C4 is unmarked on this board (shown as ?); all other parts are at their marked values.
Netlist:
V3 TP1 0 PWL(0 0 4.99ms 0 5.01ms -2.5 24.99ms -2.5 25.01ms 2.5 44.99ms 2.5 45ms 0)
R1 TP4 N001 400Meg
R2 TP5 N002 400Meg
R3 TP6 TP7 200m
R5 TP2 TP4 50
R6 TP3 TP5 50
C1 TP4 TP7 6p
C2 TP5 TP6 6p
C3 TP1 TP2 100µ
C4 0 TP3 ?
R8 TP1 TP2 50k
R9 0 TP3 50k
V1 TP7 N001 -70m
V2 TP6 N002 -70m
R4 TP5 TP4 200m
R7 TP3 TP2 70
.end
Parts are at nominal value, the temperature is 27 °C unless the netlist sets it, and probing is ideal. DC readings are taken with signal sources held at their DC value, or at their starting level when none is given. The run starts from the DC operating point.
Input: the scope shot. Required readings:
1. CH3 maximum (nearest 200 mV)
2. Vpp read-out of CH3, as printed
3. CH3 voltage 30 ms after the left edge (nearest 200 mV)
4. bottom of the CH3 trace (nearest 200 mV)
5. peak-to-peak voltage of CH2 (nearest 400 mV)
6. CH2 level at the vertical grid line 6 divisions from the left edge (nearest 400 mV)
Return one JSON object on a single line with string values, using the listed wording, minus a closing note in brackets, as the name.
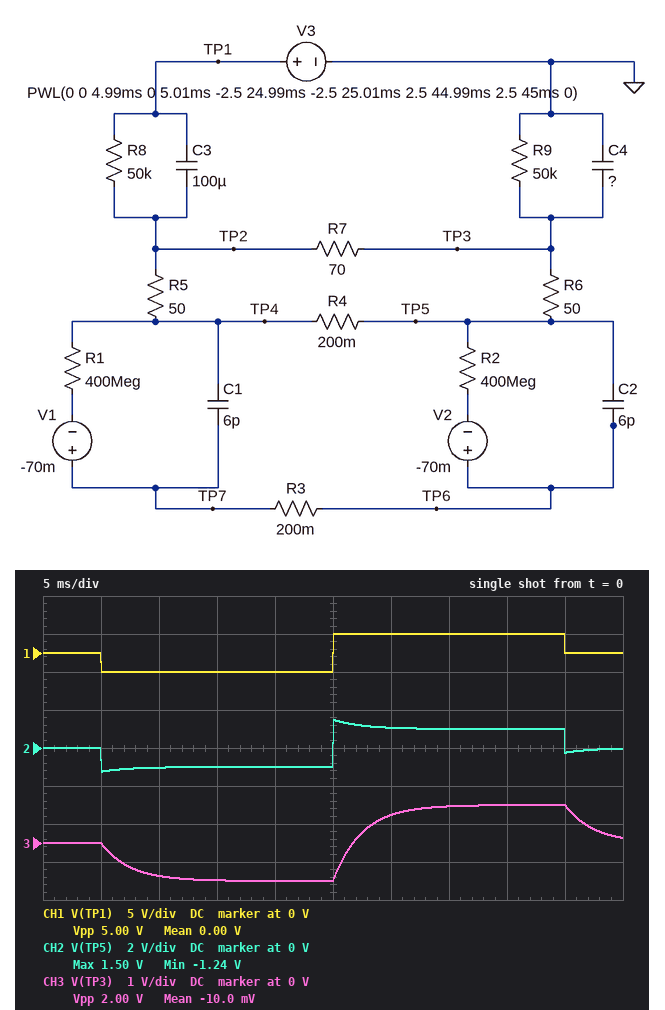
{"CH3 maximum": "1.0 V", "Vpp read-out of CH3, as printed": "2.00 V", "CH3 voltage 30 ms after the left edge": "800 mV", "bottom of the CH3 trace": "-1.0 V", "peak-to-peak voltage of CH2": "2.8 V", "CH2 level at the vertical grid line 6 divisions from the left edge": "1.2 V"}
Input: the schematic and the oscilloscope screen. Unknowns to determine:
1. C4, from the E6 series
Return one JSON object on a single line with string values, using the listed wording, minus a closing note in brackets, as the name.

{"C4, from the E6 series": "150 µF"}
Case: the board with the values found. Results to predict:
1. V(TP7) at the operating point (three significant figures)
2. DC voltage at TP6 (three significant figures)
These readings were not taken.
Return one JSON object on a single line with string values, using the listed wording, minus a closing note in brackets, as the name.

{"V(TP7) at the operating point": "-70.0 mV", "DC voltage at TP6": "-70.0 mV"}
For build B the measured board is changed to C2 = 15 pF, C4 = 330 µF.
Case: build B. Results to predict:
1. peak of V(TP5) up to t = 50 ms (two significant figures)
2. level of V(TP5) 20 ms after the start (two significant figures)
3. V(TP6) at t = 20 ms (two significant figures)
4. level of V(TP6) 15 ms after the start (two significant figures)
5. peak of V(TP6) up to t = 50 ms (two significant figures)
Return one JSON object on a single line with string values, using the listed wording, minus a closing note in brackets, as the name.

{"peak of V(TP5) up to t = 50 ms": "1.9 V", "level of V(TP5) 20 ms after the start": "-590 mV", "V(TP6) at t = 20 ms": "-660 mV", "level of V(TP6) 15 ms after the start": "-680 mV", "peak of V(TP6) up to t = 50 ms": "1.8 V"}
